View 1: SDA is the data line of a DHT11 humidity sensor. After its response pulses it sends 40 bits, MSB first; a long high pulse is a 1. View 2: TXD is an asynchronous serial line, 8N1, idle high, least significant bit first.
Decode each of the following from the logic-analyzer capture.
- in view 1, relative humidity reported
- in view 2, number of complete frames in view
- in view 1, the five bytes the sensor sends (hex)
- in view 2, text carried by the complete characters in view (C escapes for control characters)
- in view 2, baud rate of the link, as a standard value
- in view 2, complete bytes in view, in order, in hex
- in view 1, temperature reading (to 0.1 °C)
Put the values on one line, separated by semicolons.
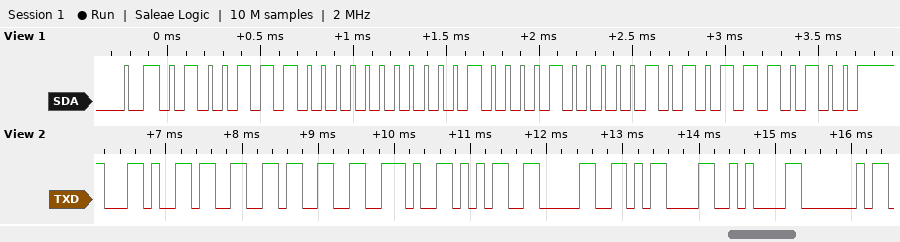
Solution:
78 %; 9; 4E 00 21 05 74; ",33.50\r\n@"; 9600 baud; 2C 33 33 2E 35 30 0D 0A 40; 33.5 °C
